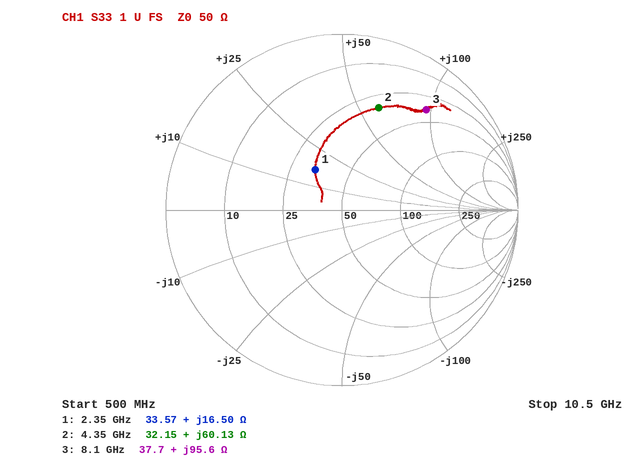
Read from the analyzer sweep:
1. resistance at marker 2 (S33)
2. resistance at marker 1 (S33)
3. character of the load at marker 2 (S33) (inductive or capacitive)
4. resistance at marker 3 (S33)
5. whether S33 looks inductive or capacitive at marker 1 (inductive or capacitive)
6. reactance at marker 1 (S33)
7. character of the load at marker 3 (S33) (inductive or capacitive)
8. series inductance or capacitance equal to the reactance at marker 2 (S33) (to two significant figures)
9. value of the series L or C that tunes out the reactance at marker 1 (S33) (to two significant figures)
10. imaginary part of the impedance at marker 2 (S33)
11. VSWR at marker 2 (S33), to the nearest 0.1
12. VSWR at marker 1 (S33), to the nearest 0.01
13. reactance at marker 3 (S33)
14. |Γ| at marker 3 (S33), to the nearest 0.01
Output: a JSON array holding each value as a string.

["32.15 Ω", "33.57 Ω", "inductive", "37.7 Ω", "inductive", "+16.50 Ω", "inductive", "2.2 nH", "4.1 pF", "+60.13 Ω", "4.2", "1.75", "+95.6 Ω", "0.74"]
